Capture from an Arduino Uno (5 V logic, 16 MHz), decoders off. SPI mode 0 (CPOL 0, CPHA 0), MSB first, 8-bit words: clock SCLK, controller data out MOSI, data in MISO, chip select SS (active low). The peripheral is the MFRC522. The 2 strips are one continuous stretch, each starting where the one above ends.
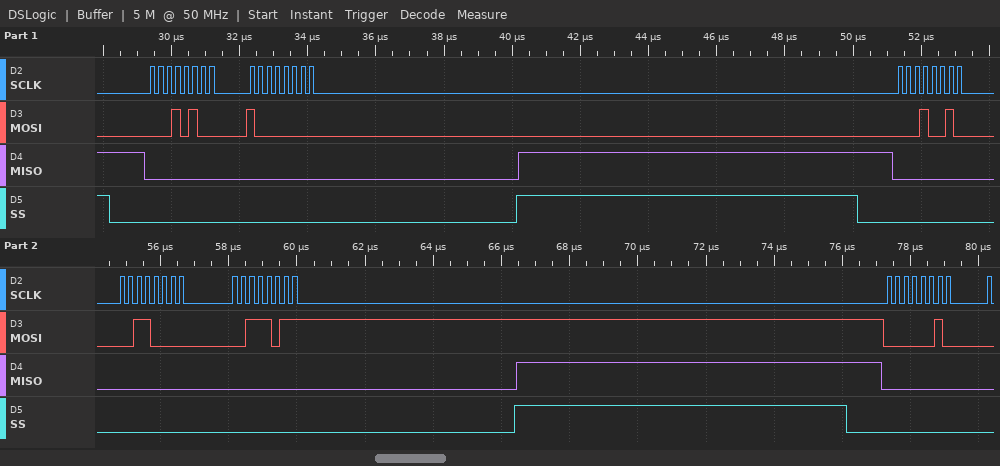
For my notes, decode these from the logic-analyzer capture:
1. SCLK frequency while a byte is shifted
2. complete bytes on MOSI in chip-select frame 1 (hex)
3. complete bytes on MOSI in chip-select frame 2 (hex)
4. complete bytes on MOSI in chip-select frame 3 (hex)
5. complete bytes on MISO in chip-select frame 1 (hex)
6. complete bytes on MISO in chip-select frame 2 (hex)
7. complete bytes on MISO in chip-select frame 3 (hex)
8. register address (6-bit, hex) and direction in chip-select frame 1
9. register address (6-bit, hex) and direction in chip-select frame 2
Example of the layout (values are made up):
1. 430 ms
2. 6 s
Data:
1. 4 MHz
2. 0x14 0x80
3. 0x12 0x30 0x3B
4. 0x02
5. 0x00 0x00
6. 0x00 0x00 0x00
7. 0x00
8. 0x0A write
9. 0x09 write
